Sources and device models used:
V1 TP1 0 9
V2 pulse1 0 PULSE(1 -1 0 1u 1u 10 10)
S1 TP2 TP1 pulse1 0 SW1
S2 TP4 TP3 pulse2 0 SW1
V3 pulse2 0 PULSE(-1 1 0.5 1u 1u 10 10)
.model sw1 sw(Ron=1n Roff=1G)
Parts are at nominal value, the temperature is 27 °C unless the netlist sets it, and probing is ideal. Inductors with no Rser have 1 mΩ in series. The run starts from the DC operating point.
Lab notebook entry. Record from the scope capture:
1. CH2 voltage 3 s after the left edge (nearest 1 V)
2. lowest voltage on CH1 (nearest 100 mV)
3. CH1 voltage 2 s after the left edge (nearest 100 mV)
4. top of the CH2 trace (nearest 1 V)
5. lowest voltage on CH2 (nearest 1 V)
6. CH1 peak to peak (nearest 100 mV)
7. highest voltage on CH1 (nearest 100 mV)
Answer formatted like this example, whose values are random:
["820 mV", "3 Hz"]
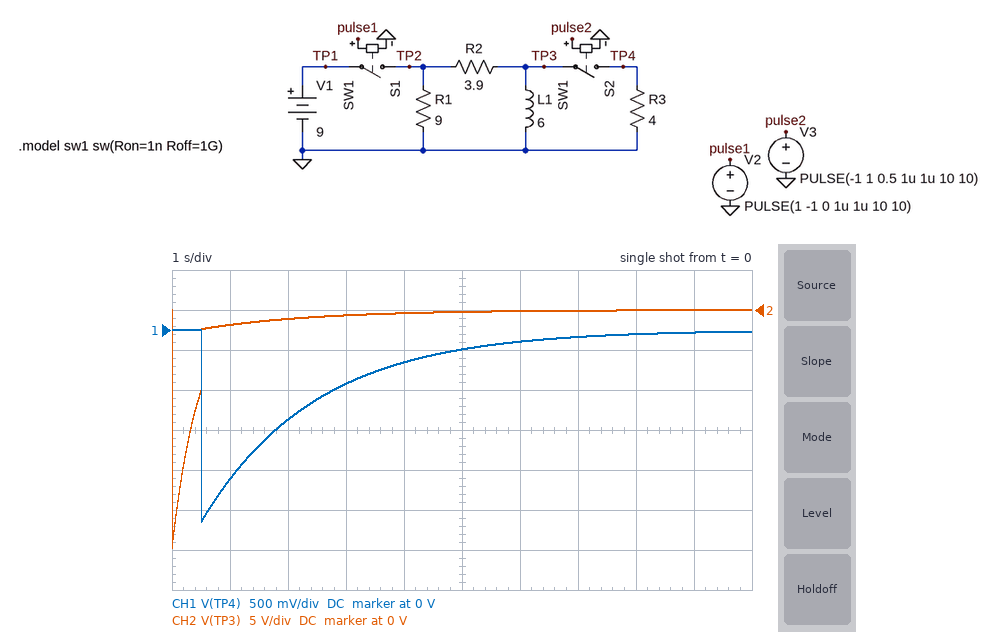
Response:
["-1 V", "-2.4 V", "-1.1 V", "0 V", "-30 V", "2.4 V", "0 V"]
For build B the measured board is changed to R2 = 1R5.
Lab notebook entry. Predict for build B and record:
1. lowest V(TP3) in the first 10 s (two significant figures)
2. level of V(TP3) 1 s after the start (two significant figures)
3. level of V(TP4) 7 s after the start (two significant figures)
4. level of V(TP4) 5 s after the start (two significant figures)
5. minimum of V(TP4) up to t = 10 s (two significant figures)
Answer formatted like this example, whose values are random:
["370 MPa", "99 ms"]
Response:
["-63 V", "-5.7 V", "-310 mV", "-820 mV", "-7.2 V"]
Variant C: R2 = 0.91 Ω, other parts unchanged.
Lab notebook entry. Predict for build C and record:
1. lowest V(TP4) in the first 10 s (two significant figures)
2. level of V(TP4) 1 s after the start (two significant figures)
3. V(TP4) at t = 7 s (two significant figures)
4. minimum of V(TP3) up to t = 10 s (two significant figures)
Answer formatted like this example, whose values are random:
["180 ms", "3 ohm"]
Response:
["-12 V", "-9.7 V", "-560 mV", "-98 V"]
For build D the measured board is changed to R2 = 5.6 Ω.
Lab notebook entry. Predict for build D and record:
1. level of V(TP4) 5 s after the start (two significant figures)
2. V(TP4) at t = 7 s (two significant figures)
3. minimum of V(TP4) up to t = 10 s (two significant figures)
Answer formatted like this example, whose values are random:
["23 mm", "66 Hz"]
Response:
["-140 mV", "-50 mV", "-1.5 V"]
